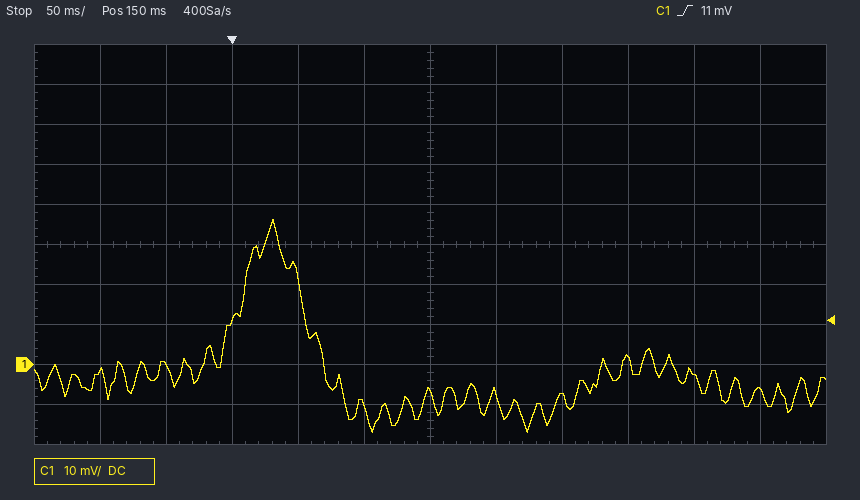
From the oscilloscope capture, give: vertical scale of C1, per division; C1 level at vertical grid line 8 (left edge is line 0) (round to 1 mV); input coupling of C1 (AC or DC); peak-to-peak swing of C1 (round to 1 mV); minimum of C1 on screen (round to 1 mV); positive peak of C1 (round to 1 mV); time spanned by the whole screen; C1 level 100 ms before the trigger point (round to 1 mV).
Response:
10 mV
-8 mV
DC
53 mV
-17 mV
36 mV
600 ms
-2 mV
